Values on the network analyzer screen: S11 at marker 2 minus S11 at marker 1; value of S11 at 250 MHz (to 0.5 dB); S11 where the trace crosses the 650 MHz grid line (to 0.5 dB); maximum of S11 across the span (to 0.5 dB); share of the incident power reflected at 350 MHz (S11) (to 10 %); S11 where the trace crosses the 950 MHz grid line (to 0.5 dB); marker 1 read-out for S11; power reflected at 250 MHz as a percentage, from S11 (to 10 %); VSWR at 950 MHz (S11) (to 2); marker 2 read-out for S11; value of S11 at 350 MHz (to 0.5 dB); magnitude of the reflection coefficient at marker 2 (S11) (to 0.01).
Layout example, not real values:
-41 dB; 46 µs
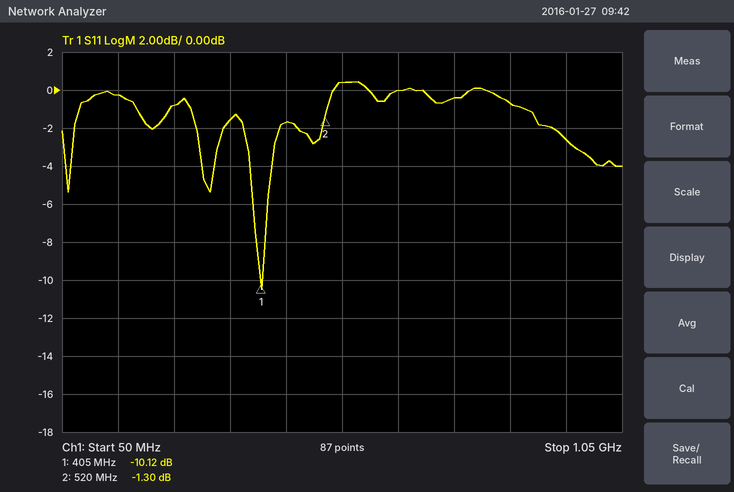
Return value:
8.82 dB; -1.0 dB; 0.0 dB; 0.5 dB; 70 %; -2.5 dB; -10.12 dB; 80 %; 6; -1.30 dB; -1.5 dB; 0.86
